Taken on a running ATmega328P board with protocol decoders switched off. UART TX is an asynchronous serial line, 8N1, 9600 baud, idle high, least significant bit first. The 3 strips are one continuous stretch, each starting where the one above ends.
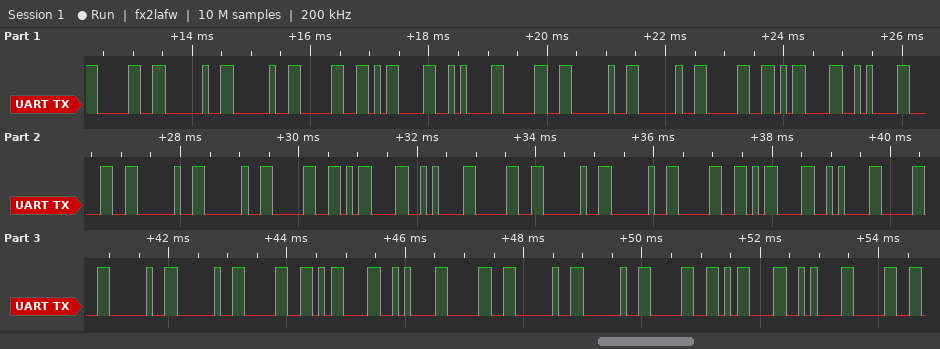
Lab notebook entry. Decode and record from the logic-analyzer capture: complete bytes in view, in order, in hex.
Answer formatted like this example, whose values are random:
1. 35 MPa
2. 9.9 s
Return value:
1. 0x30 0x20 0x20 0x30 0x0D 0x0A 0x30 0x20 0x20 0x30 0x0D 0x0A 0x30 0x20 0x20 0x30 0x0D 0x0A 0x30 0x20 0x20 0x30 0x0D 0x0A 0x30 0x20 0x20 0x30 0x0D 0x0A 0x30 0x20 0x20 0x30 0x0D 0x0A 0x30
